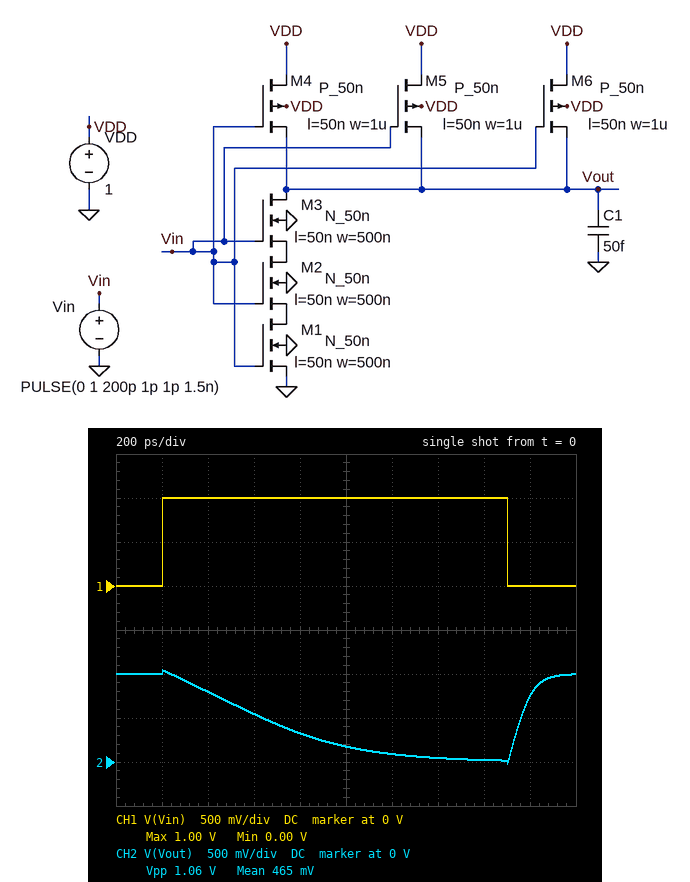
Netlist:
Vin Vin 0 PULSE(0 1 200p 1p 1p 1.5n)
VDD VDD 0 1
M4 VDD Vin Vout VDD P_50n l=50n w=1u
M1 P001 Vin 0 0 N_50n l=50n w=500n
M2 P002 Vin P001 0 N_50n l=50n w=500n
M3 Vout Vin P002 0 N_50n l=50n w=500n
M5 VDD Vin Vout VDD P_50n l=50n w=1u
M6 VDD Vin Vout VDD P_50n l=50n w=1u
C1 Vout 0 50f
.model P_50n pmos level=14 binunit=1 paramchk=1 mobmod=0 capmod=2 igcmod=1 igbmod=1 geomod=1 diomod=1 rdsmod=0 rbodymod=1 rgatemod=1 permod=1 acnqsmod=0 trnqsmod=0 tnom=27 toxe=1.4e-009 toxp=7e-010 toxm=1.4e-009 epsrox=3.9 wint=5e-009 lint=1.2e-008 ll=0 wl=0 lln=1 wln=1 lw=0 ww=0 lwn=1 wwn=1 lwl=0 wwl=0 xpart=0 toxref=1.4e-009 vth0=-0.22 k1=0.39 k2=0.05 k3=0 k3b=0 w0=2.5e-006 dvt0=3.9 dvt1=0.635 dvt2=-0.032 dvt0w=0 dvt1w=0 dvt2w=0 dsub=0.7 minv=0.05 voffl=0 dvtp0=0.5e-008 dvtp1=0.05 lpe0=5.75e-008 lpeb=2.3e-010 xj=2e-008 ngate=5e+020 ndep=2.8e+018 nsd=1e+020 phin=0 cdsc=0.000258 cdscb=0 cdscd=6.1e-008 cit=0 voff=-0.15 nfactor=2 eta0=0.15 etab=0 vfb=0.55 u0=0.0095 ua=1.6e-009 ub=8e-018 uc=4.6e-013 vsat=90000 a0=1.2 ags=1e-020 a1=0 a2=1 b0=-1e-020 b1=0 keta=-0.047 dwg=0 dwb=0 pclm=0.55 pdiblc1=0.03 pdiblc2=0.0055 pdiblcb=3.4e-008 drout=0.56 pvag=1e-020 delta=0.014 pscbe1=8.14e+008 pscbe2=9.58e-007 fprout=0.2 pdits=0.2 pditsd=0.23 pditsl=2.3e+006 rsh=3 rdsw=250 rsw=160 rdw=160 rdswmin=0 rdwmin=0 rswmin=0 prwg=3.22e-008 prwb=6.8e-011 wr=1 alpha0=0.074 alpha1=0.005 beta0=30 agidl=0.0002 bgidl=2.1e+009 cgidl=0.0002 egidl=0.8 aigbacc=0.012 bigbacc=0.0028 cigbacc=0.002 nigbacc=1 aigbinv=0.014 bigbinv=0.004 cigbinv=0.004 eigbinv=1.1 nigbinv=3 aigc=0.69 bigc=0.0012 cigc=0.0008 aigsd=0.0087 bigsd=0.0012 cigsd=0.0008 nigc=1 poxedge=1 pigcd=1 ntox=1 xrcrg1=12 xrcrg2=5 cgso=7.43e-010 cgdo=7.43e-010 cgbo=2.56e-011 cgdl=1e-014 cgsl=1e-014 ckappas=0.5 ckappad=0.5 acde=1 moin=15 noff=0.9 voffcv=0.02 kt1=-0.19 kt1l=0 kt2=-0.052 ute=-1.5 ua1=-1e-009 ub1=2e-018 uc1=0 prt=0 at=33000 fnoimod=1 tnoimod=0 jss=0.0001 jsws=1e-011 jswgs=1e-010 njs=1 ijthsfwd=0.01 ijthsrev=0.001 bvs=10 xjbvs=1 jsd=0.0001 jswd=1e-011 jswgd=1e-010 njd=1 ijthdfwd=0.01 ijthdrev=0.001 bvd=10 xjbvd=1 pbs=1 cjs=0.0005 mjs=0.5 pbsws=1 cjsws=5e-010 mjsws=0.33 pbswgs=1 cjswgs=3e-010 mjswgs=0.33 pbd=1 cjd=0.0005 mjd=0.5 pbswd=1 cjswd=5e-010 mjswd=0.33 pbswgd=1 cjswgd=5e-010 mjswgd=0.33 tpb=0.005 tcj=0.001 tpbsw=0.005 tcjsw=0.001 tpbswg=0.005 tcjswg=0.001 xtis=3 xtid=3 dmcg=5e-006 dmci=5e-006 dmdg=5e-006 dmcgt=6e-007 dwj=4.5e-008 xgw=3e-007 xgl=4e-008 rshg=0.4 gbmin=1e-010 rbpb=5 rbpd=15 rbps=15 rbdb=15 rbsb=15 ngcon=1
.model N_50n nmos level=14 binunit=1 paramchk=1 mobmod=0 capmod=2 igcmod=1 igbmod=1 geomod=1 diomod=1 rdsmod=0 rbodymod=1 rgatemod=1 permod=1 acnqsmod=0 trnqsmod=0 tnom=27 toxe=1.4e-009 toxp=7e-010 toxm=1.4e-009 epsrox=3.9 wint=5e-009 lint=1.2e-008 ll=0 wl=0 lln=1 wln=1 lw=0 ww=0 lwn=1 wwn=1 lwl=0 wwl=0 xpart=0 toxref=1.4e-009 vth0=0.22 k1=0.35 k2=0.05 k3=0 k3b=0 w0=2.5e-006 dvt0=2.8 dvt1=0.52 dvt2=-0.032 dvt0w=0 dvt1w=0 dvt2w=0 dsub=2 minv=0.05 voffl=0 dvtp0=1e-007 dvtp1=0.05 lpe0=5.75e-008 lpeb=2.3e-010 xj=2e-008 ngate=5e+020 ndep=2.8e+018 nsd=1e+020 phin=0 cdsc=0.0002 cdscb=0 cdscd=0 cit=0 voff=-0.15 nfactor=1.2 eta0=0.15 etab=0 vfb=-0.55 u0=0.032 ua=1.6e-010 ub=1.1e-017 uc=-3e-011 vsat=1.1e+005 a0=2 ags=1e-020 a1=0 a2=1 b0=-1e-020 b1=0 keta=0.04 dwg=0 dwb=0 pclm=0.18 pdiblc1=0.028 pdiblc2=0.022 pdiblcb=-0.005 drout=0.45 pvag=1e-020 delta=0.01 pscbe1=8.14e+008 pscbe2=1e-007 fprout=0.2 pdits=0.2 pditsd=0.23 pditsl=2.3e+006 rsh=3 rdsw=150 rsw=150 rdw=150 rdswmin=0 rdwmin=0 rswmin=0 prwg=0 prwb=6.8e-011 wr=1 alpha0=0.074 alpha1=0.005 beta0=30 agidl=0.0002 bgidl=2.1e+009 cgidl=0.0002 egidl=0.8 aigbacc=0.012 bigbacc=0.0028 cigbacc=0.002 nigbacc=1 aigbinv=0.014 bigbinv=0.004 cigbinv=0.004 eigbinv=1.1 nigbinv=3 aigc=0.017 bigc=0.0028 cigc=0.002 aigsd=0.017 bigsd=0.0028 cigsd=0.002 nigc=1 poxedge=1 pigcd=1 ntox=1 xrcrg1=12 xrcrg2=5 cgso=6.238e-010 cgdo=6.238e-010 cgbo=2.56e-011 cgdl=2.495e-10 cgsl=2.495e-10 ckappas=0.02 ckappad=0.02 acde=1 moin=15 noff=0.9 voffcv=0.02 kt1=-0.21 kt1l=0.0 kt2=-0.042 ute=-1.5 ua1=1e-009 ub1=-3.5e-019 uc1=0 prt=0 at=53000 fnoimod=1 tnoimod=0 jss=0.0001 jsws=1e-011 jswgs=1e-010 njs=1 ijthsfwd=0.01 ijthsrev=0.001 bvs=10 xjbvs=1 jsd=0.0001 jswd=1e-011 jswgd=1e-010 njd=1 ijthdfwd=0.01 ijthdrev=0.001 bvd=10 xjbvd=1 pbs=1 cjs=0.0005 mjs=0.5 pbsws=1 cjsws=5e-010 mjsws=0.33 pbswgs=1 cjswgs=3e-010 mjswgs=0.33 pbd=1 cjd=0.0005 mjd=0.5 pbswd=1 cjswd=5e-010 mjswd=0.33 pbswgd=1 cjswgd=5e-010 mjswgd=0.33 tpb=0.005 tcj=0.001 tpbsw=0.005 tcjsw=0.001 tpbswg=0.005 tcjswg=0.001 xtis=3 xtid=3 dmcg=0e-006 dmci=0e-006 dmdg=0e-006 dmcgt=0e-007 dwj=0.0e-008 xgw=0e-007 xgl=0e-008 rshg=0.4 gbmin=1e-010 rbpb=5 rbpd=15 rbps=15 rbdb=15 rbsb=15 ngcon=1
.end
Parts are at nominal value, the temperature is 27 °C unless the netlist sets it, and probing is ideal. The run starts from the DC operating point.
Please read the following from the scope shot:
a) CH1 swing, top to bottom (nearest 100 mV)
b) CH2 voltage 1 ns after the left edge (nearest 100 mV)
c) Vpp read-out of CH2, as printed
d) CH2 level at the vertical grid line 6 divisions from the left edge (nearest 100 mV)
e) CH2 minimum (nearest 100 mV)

1.0 V
200 mV
1.06 V
100 mV
0 V
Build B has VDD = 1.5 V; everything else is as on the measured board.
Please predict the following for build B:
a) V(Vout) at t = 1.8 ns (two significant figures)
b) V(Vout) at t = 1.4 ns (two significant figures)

1.5 V
1.2 V
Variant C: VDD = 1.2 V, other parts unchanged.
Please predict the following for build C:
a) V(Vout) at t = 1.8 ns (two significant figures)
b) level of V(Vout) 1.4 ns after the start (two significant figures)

960 mV
82 mV
